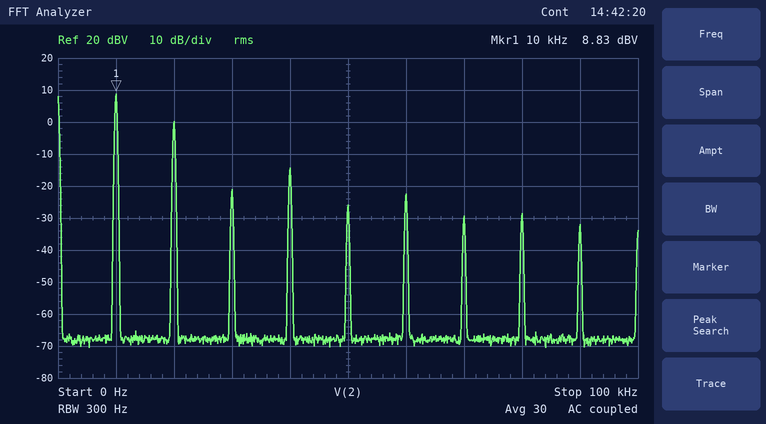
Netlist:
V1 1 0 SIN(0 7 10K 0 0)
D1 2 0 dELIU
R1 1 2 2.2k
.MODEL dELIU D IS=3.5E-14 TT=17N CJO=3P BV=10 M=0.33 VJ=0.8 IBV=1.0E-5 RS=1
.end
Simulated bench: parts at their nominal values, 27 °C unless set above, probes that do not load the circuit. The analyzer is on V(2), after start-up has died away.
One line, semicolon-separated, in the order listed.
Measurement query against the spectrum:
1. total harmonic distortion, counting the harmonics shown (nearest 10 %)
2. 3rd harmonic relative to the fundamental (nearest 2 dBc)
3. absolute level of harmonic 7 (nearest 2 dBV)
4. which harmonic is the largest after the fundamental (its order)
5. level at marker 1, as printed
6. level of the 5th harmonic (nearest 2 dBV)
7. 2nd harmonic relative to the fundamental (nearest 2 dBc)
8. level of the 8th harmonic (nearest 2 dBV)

40 %; -30 dBc; -30 dBV; 2; 8.83 dBV; -26 dBV; -8 dBc; -28 dBV
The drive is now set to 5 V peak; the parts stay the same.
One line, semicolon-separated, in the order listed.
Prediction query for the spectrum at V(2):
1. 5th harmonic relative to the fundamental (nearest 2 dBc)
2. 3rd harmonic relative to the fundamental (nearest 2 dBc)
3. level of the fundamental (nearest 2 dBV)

-32 dBc; -28 dBc; 6 dBV
